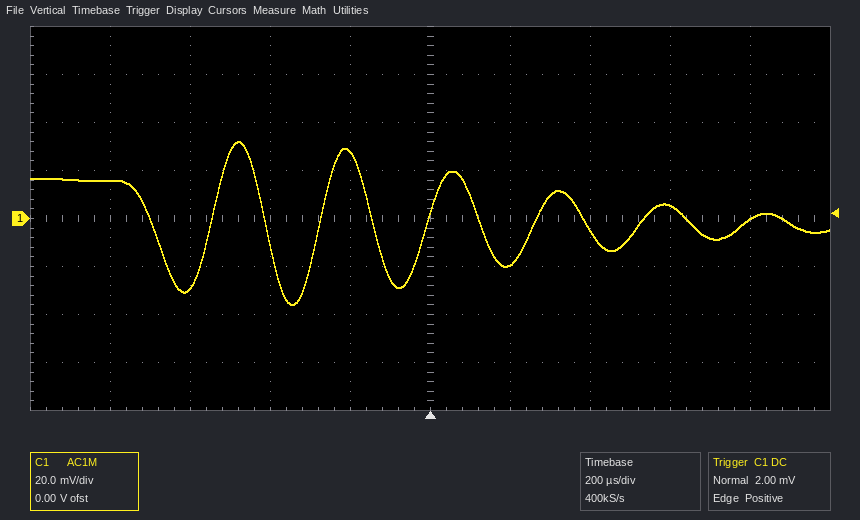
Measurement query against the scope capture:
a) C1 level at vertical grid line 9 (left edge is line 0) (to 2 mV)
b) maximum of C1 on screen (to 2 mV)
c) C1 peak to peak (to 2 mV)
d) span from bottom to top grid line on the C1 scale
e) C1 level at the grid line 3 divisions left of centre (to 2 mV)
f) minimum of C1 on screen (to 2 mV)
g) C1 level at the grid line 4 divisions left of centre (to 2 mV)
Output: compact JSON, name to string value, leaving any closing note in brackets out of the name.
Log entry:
{"C1 level at vertical grid line 9 (left edge is line 0)": "0 mV", "maximum of C1 on screen": "32 mV", "C1 peak to peak": "68 mV", "span from bottom to top grid line on the C1 scale": "160 mV", "C1 level at the grid line 3 divisions left of centre": "-28 mV", "minimum of C1 on screen": "-36 mV", "C1 level at the grid line 4 divisions left of centre": "16 mV"}
